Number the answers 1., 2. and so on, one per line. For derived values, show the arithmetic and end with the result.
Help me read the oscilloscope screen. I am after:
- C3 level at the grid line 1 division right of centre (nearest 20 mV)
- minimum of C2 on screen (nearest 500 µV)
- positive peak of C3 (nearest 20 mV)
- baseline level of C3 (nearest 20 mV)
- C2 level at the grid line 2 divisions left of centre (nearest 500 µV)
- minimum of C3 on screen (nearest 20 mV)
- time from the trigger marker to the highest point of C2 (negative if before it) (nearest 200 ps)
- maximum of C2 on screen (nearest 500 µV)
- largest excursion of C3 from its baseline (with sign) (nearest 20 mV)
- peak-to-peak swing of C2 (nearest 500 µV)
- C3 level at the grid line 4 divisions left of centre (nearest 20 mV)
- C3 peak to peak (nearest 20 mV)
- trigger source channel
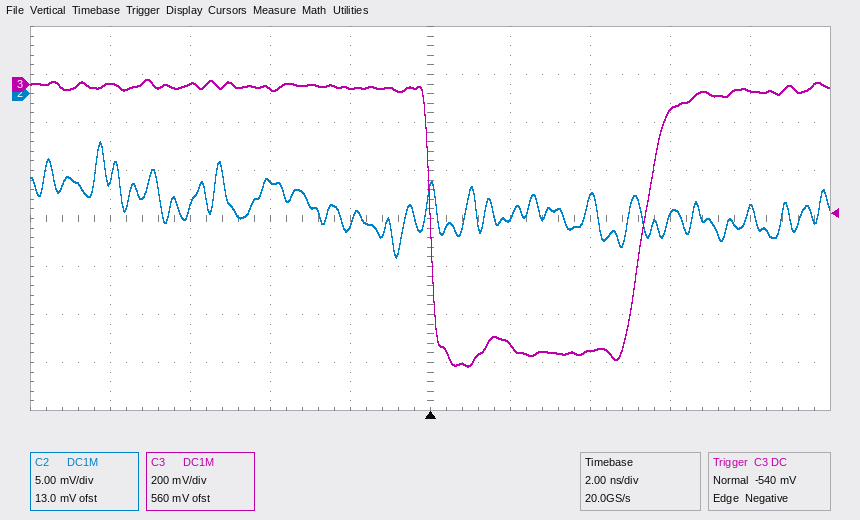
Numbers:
1. -1.08 V
2. -17.0 mV
3. 20 mV
4. -20 mV
5. -9.0 mV
6. -1.18 V
7. -8.2 ns
8. -5.0 mV
9. -1.18 V − (-20 mV) = -1.16 V
10. -5.0 mV − (-17.0 mV) = 12.0 mV
11. 0 mV
12. 20 mV − (-1.18 V) = 1.20 V
13. C3
